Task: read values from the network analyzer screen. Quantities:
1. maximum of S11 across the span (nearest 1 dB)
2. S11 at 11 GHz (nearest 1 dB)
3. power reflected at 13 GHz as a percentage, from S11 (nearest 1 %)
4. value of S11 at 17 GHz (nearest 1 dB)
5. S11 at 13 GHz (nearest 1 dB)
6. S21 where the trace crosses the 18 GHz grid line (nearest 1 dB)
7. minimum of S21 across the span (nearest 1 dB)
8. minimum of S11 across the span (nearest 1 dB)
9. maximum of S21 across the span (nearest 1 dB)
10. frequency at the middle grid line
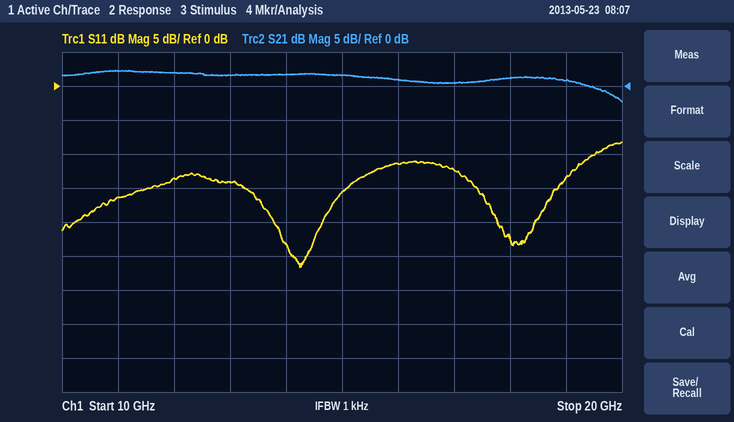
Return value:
-8 dB
-16 dB
4 %
-12 dB
-14 dB
1 dB
-2 dB
-27 dB
2 dB
15 GHz
